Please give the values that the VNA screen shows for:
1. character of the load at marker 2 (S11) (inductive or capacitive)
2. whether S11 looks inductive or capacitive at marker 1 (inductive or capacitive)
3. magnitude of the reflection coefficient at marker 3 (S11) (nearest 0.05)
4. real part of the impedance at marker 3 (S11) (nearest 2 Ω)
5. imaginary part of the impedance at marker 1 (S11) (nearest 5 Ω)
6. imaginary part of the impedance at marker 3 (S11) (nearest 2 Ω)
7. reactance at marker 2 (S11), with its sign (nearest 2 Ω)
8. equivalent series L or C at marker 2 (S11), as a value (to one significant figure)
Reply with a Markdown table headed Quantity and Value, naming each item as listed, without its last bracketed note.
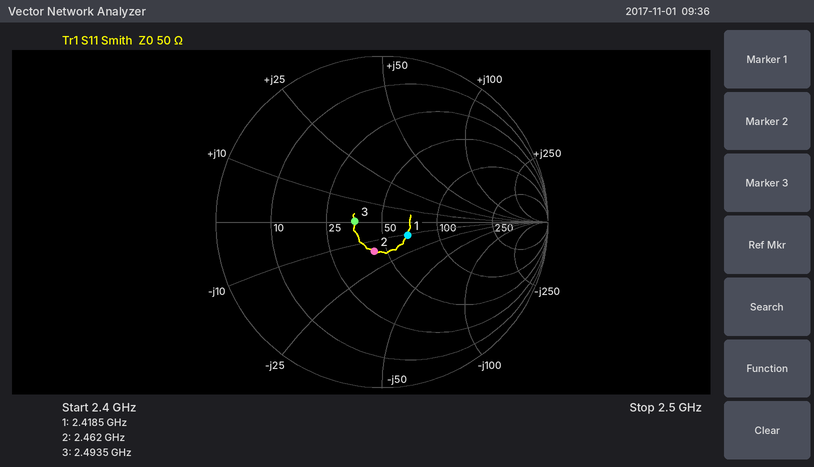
| Quantity | Value |
|---|---|
| character of the load at marker 2 (S11) | capacitive |
| whether S11 looks inductive or capacitive at marker 1 | capacitive |
| magnitude of the reflection coefficient at marker 3 (S11) | 0.15 |
| real part of the impedance at marker 3 (S11) | 36 Ω |
| imaginary part of the impedance at marker 1 (S11) | -10 Ω |
| imaginary part of the impedance at marker 3 (S11) | 0 Ω |
| reactance at marker 2 (S11), with its sign | -16 Ω |
| equivalent series L or C at marker 2 (S11), as a value | 4 pF |
